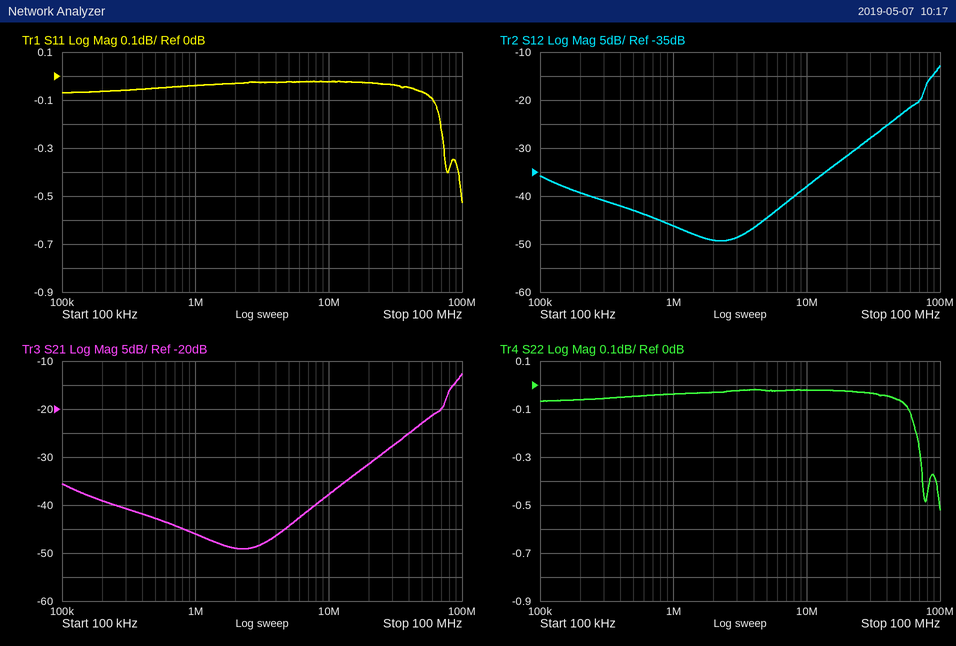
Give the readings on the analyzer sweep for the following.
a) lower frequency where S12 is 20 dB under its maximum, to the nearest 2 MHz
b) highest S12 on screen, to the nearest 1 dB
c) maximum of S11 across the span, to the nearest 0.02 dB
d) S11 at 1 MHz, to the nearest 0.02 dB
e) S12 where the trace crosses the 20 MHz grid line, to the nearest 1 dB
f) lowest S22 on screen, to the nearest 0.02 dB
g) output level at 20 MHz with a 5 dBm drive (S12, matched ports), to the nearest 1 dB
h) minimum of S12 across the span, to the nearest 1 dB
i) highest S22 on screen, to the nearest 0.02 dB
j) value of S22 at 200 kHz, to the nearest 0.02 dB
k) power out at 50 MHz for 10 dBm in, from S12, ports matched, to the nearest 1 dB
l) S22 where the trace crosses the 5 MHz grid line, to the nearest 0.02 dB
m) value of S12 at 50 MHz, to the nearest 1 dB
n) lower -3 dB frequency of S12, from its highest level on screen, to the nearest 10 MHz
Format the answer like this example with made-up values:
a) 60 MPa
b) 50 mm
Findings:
a) 18 MHz
b) -13 dB
c) -0.02 dB
d) -0.04 dB
e) -32 dB
f) -0.52 dB
g) -27 dBm
h) -49 dB
i) -0.02 dB
j) -0.06 dB
k) -13 dBm
l) -0.02 dB
m) -23 dB
n) 80 MHz
